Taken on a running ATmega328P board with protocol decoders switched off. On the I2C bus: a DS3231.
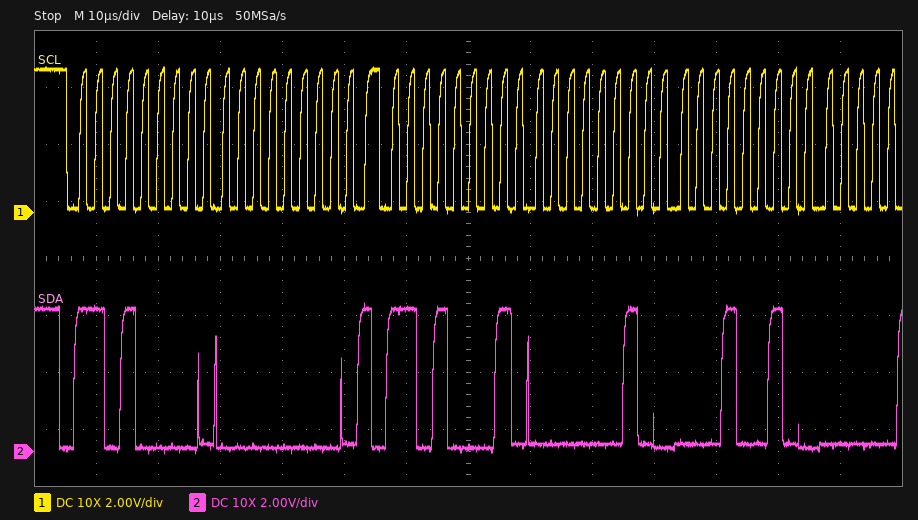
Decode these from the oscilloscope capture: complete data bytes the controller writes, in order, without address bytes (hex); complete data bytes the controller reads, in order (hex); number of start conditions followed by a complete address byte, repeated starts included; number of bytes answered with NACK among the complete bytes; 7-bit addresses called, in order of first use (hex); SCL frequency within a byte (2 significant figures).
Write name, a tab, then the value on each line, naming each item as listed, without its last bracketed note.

complete data bytes the controller writes, in order, without address bytes	00
complete data bytes the controller reads, in order	02 12
number of start conditions followed by a complete address byte, repeated starts included	2
number of bytes answered with NACK among the complete bytes	0
7-bit addresses called, in order of first use	0x68
SCL frequency within a byte	400 kHz
